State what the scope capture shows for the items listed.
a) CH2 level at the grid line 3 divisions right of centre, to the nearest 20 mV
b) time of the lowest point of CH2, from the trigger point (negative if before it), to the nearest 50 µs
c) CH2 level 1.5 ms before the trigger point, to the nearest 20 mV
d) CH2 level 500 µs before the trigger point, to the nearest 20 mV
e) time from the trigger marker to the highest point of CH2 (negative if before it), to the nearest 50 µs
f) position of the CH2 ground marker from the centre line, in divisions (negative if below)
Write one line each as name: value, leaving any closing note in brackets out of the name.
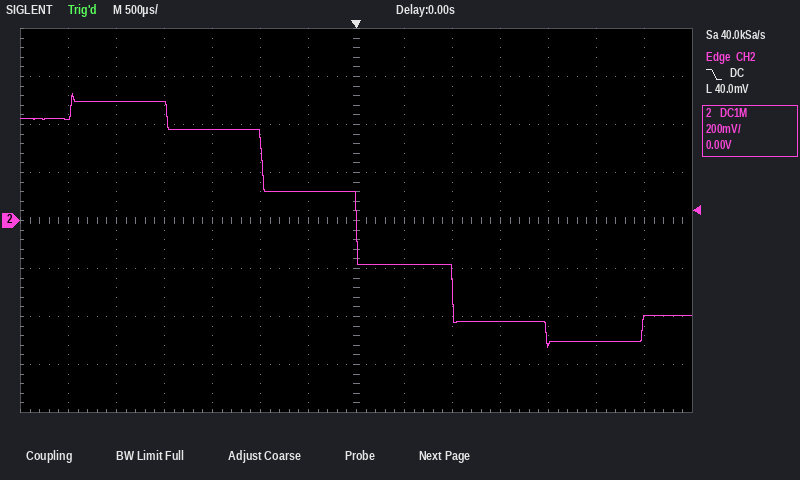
CH2 level at the grid line 3 divisions right of centre, to the nearest 20 mV: -420 mV
time of the lowest point of CH2, from the trigger point (negative if before it), to the nearest 50 µs: +2.00 ms
CH2 level 1.5 ms before the trigger point, to the nearest 20 mV: 380 mV
CH2 level 500 µs before the trigger point, to the nearest 20 mV: 120 mV
time from the trigger marker to the highest point of CH2 (negative if before it), to the nearest 50 µs: -2.95 ms
position of the CH2 ground marker from the centre line, in divisions: 0.0 div
